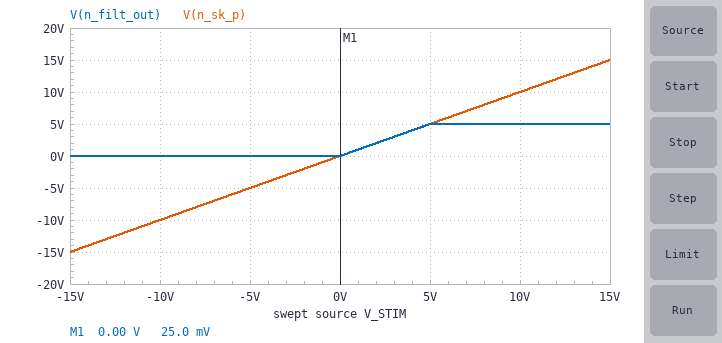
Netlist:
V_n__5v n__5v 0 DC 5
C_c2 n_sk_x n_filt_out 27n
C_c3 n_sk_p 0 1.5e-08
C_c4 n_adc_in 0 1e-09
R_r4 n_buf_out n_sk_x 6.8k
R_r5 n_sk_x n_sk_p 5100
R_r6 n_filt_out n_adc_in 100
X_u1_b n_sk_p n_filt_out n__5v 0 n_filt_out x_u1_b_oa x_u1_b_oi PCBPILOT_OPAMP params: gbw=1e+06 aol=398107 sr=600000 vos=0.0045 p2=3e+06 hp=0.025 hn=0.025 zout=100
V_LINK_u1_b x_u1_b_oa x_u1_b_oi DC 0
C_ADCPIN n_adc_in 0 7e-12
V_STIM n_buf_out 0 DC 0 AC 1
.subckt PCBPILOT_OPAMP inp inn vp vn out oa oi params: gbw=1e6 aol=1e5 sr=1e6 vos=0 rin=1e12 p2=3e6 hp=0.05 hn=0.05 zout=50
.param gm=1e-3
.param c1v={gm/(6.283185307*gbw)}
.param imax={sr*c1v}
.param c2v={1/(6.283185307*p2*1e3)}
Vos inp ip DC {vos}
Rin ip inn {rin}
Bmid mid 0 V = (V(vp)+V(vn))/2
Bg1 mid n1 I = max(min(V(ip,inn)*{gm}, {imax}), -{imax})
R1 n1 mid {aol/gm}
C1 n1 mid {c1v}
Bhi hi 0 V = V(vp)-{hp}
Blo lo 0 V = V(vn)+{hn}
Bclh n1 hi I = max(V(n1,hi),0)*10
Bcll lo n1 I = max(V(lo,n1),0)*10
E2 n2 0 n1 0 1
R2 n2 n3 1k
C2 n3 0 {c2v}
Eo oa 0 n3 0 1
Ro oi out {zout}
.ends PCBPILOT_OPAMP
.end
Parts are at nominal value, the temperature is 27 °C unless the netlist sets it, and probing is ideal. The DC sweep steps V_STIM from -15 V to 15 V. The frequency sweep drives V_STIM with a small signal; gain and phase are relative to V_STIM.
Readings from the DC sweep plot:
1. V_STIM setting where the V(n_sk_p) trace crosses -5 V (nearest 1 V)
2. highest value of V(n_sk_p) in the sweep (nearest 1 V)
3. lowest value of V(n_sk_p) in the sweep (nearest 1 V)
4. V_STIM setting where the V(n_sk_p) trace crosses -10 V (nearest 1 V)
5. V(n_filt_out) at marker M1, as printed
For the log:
-5 V
15 V
-15 V
-10 V
25.0 mV
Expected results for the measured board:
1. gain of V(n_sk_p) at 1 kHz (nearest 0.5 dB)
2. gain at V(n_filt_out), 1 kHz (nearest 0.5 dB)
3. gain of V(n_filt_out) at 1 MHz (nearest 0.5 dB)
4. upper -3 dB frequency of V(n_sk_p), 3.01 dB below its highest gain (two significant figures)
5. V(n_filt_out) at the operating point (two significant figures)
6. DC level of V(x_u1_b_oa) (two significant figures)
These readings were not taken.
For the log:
-7.5 dB
-42.0 dB
-39.5 dB
490 Hz
25 mV
25 mV
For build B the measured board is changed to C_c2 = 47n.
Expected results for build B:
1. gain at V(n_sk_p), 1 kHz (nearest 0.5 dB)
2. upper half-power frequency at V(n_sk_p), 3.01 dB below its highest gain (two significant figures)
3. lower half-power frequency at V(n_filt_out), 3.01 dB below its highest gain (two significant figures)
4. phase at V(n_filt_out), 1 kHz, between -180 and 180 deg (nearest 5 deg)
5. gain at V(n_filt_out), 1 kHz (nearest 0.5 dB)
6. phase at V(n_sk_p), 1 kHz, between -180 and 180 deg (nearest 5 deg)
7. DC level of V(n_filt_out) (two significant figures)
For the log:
-10.0 dB
350 Hz
850 Hz
25 deg
-39.5 dB
-90 deg
25 mV
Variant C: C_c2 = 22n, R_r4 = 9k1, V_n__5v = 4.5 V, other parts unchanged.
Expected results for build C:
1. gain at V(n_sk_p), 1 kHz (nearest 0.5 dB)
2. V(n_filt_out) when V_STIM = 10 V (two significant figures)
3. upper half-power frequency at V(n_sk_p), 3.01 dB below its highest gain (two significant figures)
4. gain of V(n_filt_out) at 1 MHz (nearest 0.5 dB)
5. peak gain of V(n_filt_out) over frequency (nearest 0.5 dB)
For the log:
-8.5 dB
4.5 V
420 Hz
-42.0 dB
-39.5 dB
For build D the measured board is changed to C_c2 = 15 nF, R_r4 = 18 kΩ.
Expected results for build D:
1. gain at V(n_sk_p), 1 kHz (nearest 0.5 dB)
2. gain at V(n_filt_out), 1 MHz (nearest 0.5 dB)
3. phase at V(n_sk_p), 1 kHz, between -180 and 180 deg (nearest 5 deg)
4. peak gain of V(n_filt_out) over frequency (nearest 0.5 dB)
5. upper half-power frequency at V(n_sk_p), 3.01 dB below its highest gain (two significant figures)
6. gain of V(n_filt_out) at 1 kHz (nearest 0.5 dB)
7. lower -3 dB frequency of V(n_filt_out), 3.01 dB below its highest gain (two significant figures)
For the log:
-12.0 dB
-48.0 dB
-85 deg
-45.5 dB
270 Hz
-51.5 dB
3.2 kHz
